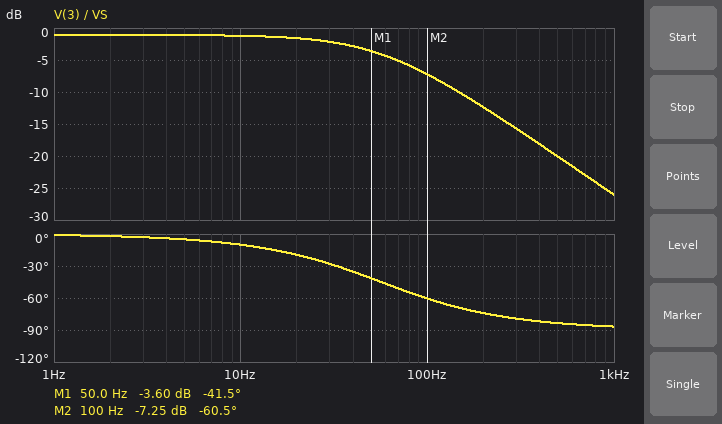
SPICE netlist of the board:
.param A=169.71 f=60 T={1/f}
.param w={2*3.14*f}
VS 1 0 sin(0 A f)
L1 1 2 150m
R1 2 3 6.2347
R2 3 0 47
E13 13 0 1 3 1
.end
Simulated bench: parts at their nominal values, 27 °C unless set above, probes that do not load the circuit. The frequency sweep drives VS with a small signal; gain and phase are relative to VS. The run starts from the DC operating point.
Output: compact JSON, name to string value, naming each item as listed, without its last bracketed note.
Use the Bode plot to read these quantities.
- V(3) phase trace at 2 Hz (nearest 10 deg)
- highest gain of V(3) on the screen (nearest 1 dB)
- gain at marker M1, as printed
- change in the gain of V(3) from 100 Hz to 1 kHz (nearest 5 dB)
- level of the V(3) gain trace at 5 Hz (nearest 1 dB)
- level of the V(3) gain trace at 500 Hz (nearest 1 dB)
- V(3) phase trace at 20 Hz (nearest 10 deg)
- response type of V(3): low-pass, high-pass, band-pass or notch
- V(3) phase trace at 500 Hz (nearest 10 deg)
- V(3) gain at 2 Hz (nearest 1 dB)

{"V(3) phase trace at 2 Hz": "0 deg", "highest gain of V(3) on the screen": "-1 dB", "gain at marker M1, as printed": "-3.60 dB", "change in the gain of V(3) from 100 Hz to 1 kHz": "-20 dB", "level of the V(3) gain trace at 5 Hz": "-1 dB", "level of the V(3) gain trace at 500 Hz": "-20 dB", "V(3) phase trace at 20 Hz": "-20 deg", "response type of V(3): low-pass, high-pass, band-pass or notch": "low-pass", "V(3) phase trace at 500 Hz": "-80 deg", "V(3) gain at 2 Hz": "-1 dB"}
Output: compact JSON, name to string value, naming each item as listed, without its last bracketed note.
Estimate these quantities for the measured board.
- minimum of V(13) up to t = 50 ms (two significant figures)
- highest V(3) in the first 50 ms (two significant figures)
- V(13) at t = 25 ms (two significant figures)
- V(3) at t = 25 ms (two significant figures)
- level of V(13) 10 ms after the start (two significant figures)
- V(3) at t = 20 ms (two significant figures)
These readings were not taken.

{"minimum of V(13) up to t = 50 ms": "-130 V", "highest V(3) in the first 50 ms": "110 V", "V(13) at t = 25 ms": "-75 V", "V(3) at t = 25 ms": "75 V", "level of V(13) 10 ms after the start": "-120 V", "V(3) at t = 20 ms": "44 V"}
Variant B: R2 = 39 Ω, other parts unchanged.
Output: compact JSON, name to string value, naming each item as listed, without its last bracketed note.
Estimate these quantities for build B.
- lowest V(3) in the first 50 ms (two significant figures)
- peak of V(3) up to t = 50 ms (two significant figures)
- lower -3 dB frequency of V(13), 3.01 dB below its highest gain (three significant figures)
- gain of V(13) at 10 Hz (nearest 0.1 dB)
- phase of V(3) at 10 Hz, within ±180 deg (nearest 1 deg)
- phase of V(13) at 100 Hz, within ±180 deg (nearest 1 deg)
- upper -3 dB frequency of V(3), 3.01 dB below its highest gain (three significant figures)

{"lowest V(3) in the first 50 ms": "-91 V", "peak of V(3) up to t = 50 ms": "100 V", "lower -3 dB frequency of V(13), 3.01 dB below its highest gain": "47.1 Hz", "gain of V(13) at 10 Hz": "-12.2 dB", "phase of V(3) at 10 Hz, within ±180 deg": "-12 deg", "phase of V(13) at 100 Hz, within ±180 deg": "22 deg", "upper -3 dB frequency of V(3), 3.01 dB below its highest gain": "48.0 Hz"}
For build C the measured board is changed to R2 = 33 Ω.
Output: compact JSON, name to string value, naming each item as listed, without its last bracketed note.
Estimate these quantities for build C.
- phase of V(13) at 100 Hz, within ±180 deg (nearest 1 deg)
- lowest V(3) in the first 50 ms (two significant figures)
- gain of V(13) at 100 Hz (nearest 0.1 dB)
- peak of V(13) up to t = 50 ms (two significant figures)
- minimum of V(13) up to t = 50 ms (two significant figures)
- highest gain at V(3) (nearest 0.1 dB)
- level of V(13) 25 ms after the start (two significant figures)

{"phase of V(13) at 100 Hz, within ±180 deg": "19 deg", "lowest V(3) in the first 50 ms": "-81 V", "gain of V(13) at 100 Hz": "-0.7 dB", "peak of V(13) up to t = 50 ms": "140 V", "minimum of V(13) up to t = 50 ms": "-140 V", "highest gain at V(3)": "-1.5 dB", "level of V(13) 25 ms after the start": "-67 V"}
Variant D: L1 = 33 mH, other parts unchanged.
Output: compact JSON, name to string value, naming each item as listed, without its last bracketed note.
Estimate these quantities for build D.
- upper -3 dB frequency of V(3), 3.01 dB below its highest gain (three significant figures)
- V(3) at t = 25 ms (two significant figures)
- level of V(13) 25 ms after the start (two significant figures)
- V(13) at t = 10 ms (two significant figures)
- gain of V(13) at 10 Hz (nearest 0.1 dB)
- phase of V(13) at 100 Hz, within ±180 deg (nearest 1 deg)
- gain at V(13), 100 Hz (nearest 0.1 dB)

{"upper -3 dB frequency of V(3), 3.01 dB below its highest gain": "257 Hz", "V(3) at t = 25 ms": "33 V", "level of V(13) 25 ms after the start": "-33 V", "V(13) at t = 10 ms": "-43 V", "gain of V(13) at 10 Hz": "-18.2 dB", "phase of V(13) at 100 Hz, within ±180 deg": "52 deg", "gain at V(13), 100 Hz": "-8.4 dB"}
